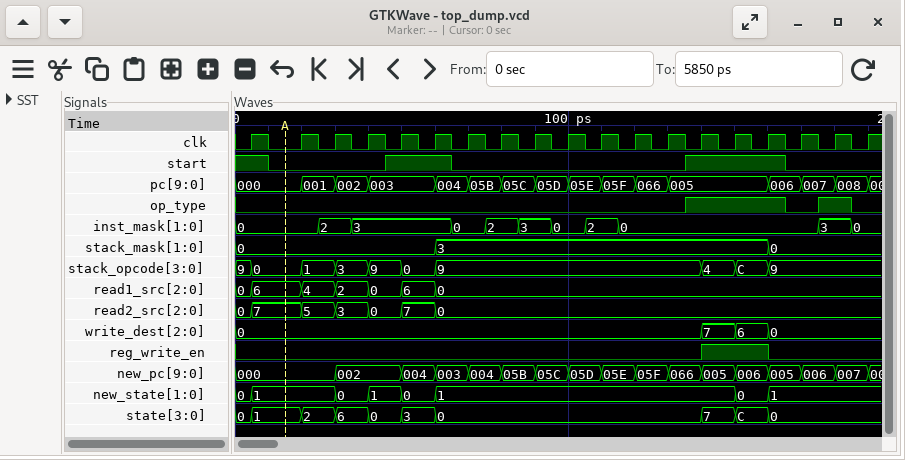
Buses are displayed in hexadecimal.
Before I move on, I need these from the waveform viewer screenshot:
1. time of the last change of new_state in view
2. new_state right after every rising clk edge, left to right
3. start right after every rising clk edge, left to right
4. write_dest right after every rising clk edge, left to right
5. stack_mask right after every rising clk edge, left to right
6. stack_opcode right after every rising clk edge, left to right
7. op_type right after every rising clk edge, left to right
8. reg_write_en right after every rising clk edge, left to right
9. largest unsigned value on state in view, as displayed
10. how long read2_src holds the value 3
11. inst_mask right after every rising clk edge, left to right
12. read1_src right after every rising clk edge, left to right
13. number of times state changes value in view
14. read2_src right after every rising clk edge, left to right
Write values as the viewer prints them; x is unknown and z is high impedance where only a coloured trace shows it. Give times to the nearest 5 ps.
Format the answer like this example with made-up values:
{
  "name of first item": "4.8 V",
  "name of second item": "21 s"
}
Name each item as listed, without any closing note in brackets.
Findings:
{
  "time of the last change of new_state in view": "160 ps",
  "new_state right after every rising clk edge, left to right": "1, 1, 0, 1, 0, 1, 1, 1, 1, 1, 1, 1, 1, 1, 0, 1, 1, 1, 1",
  "start right after every rising clk edge, left to right": "1 0 0 0 1 1 0 0 0 0 0 0 0 1 1 1 0 0 0",
  "write_dest right after every rising clk edge, left to right": "0, 0, 0, 0, 0, 0, 0, 0, 0, 0, 0, 0, 0, 7, 6, 0, 0, 0, 0",
  "stack_mask right after every rising clk edge, left to right": "0, 0, 0, 0, 0, 3, 3, 3, 3, 3, 3, 3, 3, 3, 3, 0, 0, 0, 0",
  "stack_opcode right after every rising clk edge, left to right": "0, 1, 3, 9, 0, 9, 9, 9, 9, 9, 9, 9, 9, 4, C, 9, 9, 9, 9",
  "op_type right after every rising clk edge, left to right": "0 0 0 0 0 0 0 0 0 0 0 0 0 1 1 1 0 1 0",
  "reg_write_en right after every rising clk edge, left to right": "0 0 0 0 0 0 0 0 0 0 0 0 0 1 1 0 0 0 0",
  "largest unsigned value on state in view, as displayed": "C",
  "how long read2_src holds the value 3": "10 ps",
  "inst_mask right after every rising clk edge, left to right": "0, 0, 2, 3, 3, 3, 0, 2, 3, 0, 2, 0, 0, 0, 0, 0, 0, 3, 0",
  "read1_src right after every rising clk edge, left to right": "6, 4, 2, 0, 6, 0, 0, 0, 0, 0, 0, 0, 0, 0, 0, 0, 0, 0, 0",
  "number of times state changes value in view": "9",
  "read2_src right after every rising clk edge, left to right": "7, 5, 3, 0, 7, 0, 0, 0, 0, 0, 0, 0, 0, 0, 0, 0, 0, 0, 0"
}
